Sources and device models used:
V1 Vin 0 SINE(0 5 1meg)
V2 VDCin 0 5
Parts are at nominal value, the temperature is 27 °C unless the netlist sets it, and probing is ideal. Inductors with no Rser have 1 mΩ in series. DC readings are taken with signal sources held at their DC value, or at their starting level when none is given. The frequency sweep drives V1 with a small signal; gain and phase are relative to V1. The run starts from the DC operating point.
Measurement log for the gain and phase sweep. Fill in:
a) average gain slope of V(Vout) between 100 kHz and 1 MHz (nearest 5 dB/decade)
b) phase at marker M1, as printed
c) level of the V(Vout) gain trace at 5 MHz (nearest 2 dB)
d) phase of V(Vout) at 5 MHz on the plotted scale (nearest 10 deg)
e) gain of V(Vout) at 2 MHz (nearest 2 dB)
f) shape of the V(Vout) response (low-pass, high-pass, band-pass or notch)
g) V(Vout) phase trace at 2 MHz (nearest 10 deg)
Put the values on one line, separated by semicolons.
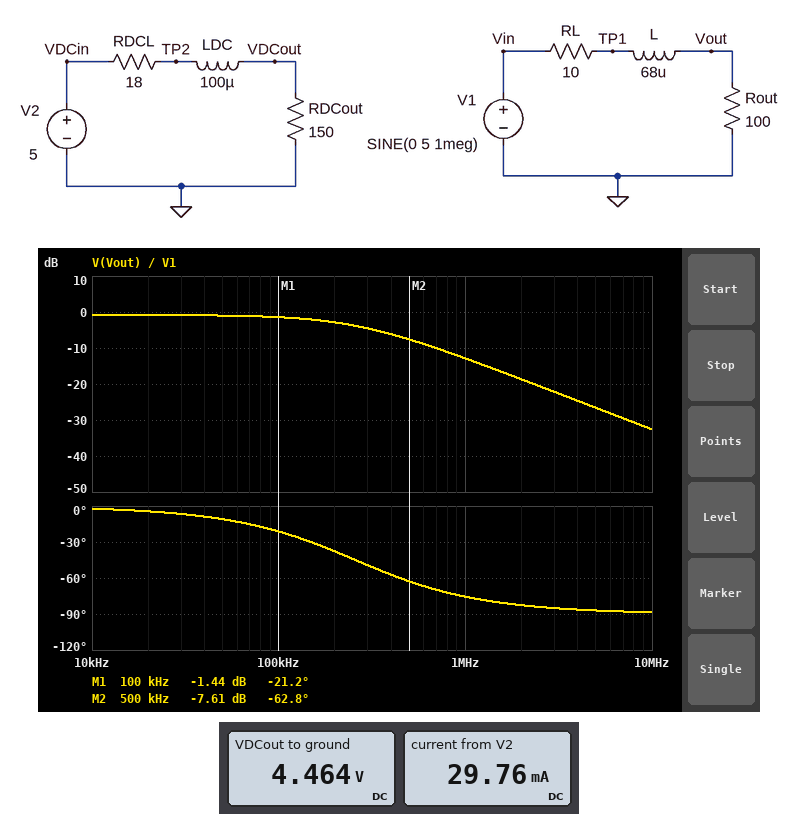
-10 dB/decade; -21.2 deg; -26 dB; -90 deg; -18 dB; low-pass; -80 deg
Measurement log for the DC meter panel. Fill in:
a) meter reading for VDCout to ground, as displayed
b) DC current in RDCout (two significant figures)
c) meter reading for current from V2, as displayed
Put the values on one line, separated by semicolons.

4.464 V; 30 mA; 29.76 mA
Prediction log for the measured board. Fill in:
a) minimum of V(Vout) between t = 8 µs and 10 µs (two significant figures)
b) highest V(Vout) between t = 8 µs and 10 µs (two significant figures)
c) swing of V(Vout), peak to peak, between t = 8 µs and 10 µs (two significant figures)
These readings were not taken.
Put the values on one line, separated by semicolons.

-1.1 V; 1.1 V; 2.3 V
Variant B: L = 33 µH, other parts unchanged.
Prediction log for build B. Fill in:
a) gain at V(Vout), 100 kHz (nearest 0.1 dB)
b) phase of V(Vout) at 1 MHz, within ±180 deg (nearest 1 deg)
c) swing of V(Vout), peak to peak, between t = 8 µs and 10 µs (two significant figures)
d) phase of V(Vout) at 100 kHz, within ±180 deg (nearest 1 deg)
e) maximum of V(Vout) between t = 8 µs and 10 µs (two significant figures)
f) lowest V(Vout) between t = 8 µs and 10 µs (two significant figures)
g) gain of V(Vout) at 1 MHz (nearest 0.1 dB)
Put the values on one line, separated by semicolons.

-1.0 dB; -62 deg; 4.3 V; -11 deg; 2.1 V; -2.1 V; -7.4 dB
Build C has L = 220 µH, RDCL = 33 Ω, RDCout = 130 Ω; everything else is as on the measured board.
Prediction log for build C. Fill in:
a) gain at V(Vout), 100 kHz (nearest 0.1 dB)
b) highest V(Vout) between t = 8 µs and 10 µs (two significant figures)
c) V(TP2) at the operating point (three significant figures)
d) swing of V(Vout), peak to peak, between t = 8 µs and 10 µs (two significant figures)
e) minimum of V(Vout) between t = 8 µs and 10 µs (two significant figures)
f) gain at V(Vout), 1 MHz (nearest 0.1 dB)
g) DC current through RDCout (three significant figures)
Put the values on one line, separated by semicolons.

-4.9 dB; 370 mV; 3.99 V; 720 mV; -360 mV; -22.8 dB; 30.7 mA
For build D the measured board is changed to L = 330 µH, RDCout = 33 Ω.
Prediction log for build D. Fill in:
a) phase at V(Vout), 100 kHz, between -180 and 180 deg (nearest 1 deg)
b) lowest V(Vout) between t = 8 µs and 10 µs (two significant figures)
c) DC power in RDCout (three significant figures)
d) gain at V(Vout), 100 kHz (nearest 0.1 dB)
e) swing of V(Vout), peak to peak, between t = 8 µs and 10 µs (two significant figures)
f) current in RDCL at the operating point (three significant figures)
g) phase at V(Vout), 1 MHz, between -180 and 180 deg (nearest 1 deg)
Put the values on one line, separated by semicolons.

-62 deg; -230 mV; 317 mW; -7.4 dB; 490 mV; 98.0 mA; -87 deg
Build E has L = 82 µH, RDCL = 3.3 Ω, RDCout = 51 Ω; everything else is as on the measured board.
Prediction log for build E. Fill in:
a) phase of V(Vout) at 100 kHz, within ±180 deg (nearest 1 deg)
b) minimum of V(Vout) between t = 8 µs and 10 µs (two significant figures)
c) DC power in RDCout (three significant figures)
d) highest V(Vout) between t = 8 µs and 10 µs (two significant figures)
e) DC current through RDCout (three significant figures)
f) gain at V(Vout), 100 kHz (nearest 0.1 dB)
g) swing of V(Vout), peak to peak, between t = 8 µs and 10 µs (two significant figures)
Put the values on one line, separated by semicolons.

-25 deg; -950 mV; 432 mW; 950 mV; 92.1 mA; -1.7 dB; 1.9 V
